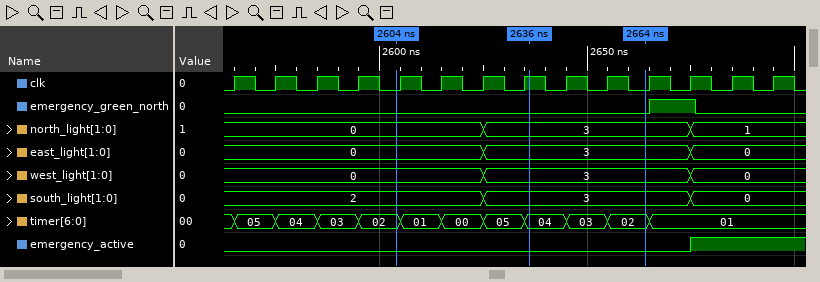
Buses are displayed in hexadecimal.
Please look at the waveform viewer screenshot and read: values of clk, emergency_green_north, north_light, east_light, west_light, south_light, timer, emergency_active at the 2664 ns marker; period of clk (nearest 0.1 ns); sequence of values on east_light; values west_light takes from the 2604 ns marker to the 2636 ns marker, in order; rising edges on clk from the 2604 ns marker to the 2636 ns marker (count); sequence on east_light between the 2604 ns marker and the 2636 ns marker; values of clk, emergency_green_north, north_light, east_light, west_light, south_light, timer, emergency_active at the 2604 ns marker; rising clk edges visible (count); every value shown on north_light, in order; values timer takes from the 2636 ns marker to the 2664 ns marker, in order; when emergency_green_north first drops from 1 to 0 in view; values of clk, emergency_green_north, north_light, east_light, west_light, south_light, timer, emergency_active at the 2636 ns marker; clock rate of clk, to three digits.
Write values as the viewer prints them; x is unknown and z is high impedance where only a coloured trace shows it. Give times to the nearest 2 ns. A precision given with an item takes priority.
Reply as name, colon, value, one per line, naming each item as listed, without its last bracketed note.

values of clk, emergency_green_north, north_light, east_light, west_light, south_light, timer, emergency_active at the 2664 ns marker: clk=0, emergency_green_north=0, north_light=3, east_light=3, west_light=3, south_light=3, timer=02, emergency_active=0
period of clk: 10 ns
sequence of values on east_light: 0, 3, 0
values west_light takes from the 2604 ns marker to the 2636 ns marker, in order: 0, 3
rising edges on clk from the 2604 ns marker to the 2636 ns marker: 4
sequence on east_light between the 2604 ns marker and the 2636 ns marker: 0, 3
values of clk, emergency_green_north, north_light, east_light, west_light, south_light, timer, emergency_active at the 2604 ns marker: clk=0, emergency_green_north=0, north_light=0, east_light=0, west_light=0, south_light=2, timer=02, emergency_active=0
rising clk edges visible: 14
every value shown on north_light, in order: 0, 3, 1
values timer takes from the 2636 ns marker to the 2664 ns marker, in order: 04, 03, 02
when emergency_green_north first drops from 1 to 0 in view: 2676 ns
values of clk, emergency_green_north, north_light, east_light, west_light, south_light, timer, emergency_active at the 2636 ns marker: clk=1, emergency_green_north=0, north_light=3, east_light=3, west_light=3, south_light=3, timer=04, emergency_active=0
clock rate of clk, to three digits: 100 MHz
